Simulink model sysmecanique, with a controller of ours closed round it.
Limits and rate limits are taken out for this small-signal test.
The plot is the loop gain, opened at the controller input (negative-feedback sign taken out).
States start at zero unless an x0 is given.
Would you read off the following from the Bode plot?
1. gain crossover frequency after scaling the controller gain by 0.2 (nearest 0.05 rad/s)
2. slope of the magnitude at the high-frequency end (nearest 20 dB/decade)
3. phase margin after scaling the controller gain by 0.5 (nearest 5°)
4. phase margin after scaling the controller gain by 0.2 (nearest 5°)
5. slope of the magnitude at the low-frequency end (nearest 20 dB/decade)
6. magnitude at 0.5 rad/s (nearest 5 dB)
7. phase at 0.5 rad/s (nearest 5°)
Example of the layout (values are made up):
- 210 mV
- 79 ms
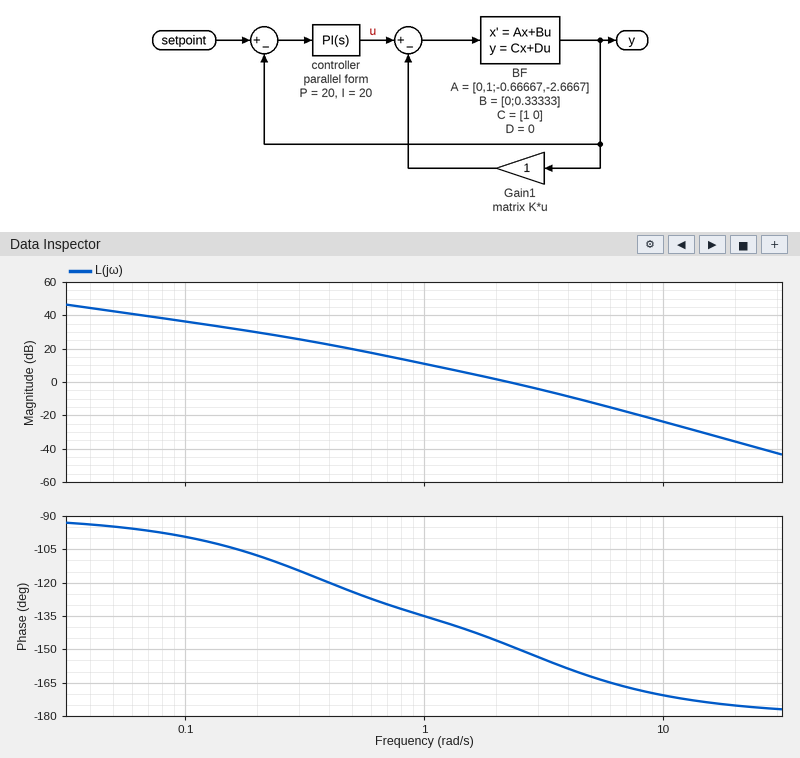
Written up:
- 0.80 rad/s
- -40 dB/decade
- 40°
- 50°
- -20 dB/decade
- 20 dB
- -125°
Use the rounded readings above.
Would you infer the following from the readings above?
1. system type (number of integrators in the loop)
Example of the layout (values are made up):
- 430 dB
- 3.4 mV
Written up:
- 1
